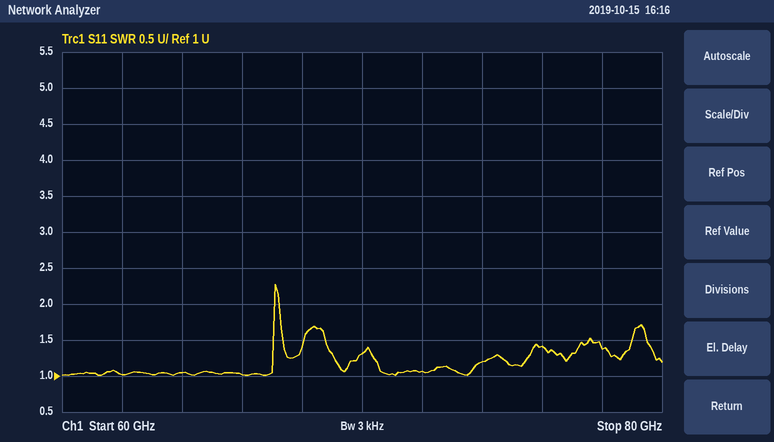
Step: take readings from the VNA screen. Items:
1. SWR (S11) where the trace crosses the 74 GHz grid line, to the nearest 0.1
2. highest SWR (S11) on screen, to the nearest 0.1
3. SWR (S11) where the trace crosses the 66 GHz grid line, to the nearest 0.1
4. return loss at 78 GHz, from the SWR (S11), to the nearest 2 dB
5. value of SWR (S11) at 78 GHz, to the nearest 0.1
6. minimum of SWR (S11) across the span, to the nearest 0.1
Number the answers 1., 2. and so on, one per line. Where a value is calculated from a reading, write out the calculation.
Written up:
1. 1.2
2. 2.3
3. 1.0
4. −20 log10((1.4 − 1)/(1.4 + 1)) ≈ 16 dB
5. 1.4
6. 1.0
